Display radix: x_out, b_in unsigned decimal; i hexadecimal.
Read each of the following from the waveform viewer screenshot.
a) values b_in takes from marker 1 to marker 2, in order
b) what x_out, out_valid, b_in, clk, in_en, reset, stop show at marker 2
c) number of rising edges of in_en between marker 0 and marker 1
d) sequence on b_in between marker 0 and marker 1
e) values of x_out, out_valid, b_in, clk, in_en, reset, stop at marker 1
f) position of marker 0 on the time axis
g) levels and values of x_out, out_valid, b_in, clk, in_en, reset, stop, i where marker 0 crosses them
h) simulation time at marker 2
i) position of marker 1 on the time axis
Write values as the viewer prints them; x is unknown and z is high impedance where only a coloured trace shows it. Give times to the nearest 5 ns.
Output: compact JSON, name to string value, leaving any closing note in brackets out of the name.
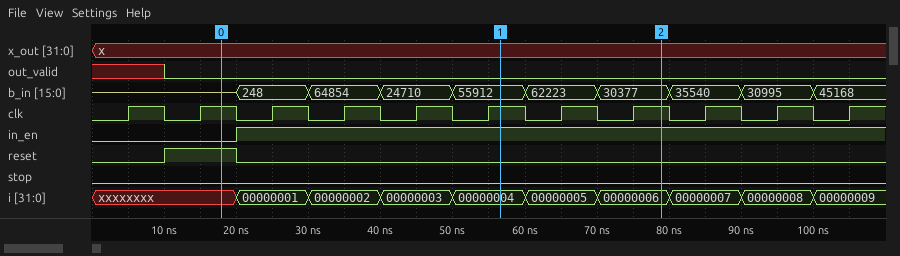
{"values b_in takes from marker 1 to marker 2, in order": "55912, 62223, 30377", "what x_out, out_valid, b_in, clk, in_en, reset, stop show at marker 2": "x_out=x, out_valid=0, b_in=30377, clk=1, in_en=1, reset=0, stop=0", "number of rising edges of in_en between marker 0 and marker 1": "1", "sequence on b_in between marker 0 and marker 1": "z, 248, 64854, 24710, 55912", "values of x_out, out_valid, b_in, clk, in_en, reset, stop at marker 1": "x_out=x, out_valid=0, b_in=55912, clk=1, in_en=1, reset=0, stop=0", "position of marker 0 on the time axis": "20 ns", "levels and values of x_out, out_valid, b_in, clk, in_en, reset, stop, i where marker 0 crosses them": "x_out=x, out_valid=0, b_in=z, clk=1, in_en=0, reset=1, stop=0, i=xxxxxxxx", "simulation time at marker 2": "80 ns", "position of marker 1 on the time axis": "55 ns"}
